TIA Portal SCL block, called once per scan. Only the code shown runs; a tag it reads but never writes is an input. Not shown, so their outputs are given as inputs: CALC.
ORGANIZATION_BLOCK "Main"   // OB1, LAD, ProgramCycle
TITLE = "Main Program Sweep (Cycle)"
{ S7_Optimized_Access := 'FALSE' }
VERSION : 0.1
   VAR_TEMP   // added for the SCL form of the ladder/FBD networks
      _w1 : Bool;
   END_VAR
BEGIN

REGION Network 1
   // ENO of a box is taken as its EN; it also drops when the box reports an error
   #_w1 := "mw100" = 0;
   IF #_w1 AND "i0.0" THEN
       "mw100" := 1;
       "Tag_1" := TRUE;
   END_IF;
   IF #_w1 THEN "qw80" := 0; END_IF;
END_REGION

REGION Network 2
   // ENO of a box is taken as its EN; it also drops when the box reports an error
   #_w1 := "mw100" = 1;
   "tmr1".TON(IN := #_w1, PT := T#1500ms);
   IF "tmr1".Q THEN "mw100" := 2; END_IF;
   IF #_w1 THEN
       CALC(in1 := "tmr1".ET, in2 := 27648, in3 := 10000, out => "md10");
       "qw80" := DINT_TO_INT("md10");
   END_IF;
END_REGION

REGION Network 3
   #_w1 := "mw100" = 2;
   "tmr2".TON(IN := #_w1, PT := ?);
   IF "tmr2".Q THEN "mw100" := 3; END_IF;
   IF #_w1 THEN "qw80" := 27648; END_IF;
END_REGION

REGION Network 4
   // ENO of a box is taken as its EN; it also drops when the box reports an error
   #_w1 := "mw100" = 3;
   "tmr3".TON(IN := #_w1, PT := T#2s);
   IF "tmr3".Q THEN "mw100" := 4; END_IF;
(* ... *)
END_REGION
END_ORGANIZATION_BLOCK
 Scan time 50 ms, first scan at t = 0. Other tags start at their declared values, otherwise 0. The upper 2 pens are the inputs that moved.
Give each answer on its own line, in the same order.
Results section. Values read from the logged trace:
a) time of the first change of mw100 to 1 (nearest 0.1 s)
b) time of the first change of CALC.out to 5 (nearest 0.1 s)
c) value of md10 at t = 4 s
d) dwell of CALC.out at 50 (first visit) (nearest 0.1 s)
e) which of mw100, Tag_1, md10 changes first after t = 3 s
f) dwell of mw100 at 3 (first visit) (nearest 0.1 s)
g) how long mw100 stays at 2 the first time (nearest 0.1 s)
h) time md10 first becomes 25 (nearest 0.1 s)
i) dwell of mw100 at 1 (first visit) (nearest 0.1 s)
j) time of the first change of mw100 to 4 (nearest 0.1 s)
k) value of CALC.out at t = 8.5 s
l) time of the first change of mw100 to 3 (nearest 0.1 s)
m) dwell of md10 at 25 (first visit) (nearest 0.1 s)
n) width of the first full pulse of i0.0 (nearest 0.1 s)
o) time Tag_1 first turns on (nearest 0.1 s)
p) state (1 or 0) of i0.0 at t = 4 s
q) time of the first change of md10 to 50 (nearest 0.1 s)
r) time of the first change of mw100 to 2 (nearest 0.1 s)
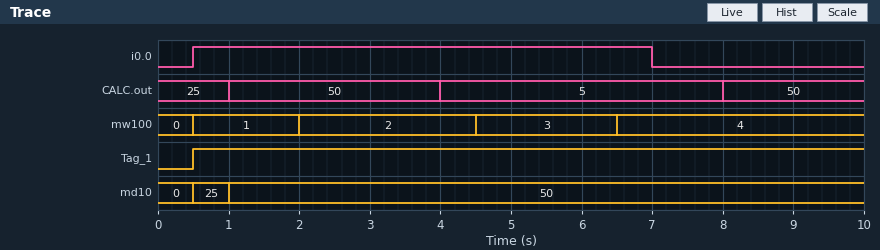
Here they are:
0.5 s
4.0 s
50
3.0 s
mw100
2.0 s
2.5 s
0.5 s
1.5 s
6.5 s
50
4.5 s
0.5 s
6.5 s
0.5 s
1
1.0 s
2.0 s
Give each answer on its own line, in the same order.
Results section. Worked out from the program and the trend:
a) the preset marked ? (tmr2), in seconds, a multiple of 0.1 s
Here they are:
2.5 s
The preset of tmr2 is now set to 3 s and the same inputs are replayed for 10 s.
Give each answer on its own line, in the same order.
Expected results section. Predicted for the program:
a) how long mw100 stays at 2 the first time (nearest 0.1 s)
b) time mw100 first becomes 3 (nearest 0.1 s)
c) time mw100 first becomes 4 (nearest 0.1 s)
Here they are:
3.0 s
5.0 s
7.0 s
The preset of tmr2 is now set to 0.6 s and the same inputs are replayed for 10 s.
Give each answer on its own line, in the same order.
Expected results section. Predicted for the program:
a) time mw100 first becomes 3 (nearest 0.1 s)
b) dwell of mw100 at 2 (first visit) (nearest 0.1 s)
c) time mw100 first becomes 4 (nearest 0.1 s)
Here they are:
2.6 s
0.6 s
4.6 s
